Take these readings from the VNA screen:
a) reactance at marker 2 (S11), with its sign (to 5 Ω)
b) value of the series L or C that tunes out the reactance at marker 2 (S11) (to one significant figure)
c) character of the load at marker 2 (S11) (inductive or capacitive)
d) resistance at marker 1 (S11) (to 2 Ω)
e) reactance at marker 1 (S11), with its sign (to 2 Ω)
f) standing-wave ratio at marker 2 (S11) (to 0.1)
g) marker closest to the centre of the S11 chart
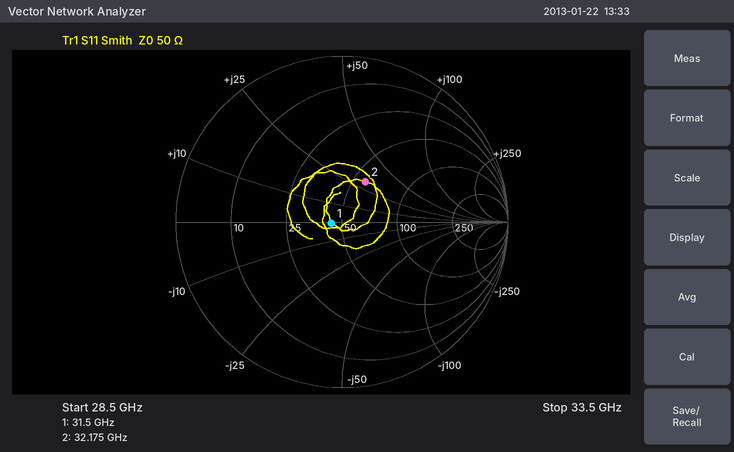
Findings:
+30 Ω
200 fF
inductive
44 Ω
0 Ω
1.8
marker 1
